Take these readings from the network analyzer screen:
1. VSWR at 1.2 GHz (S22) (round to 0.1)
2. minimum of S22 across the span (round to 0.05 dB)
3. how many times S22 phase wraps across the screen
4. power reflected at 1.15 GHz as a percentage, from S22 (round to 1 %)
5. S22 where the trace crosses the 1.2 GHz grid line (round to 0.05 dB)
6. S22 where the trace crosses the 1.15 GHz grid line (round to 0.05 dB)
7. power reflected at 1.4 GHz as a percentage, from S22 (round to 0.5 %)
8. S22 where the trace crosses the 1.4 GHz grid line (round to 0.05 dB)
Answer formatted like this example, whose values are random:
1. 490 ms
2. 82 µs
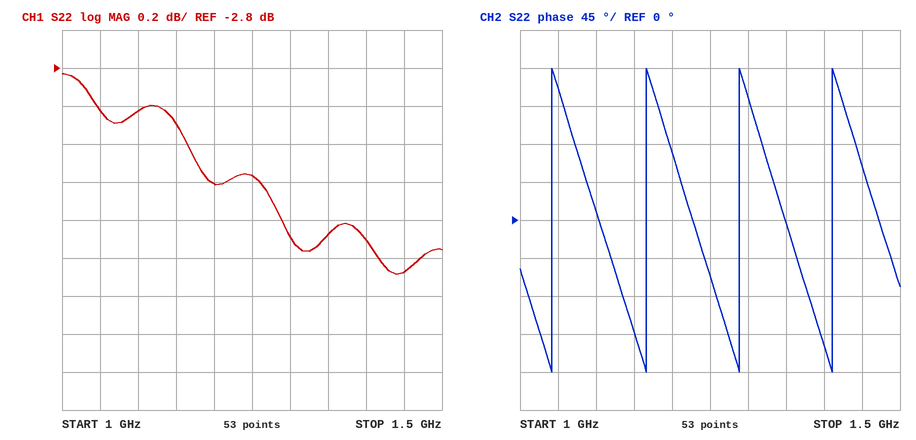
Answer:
1. 5.2
2. -3.90 dB
3. 4
4. 49 %
5. -3.40 dB
6. -3.10 dB
7. 42.5 %
8. -3.70 dB
